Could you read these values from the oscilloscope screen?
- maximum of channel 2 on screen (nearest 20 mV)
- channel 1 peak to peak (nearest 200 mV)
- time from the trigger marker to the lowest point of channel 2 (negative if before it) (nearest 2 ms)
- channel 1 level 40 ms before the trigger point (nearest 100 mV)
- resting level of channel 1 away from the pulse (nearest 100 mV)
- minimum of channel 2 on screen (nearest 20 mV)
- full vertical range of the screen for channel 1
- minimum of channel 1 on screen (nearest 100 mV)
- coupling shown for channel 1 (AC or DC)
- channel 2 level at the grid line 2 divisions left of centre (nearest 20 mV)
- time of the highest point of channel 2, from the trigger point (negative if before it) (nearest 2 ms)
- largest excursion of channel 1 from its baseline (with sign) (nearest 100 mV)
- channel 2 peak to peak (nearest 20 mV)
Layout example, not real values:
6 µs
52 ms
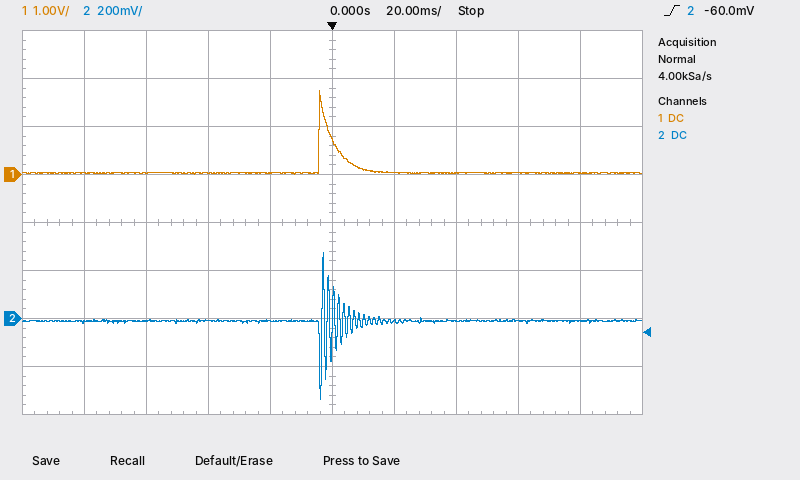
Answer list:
280 mV
1.8 V
-4 ms
0.0 V
0.0 V
-340 mV
8 V
0.0 V
DC
0 mV
-2 ms
+1.7 V
620 mV
